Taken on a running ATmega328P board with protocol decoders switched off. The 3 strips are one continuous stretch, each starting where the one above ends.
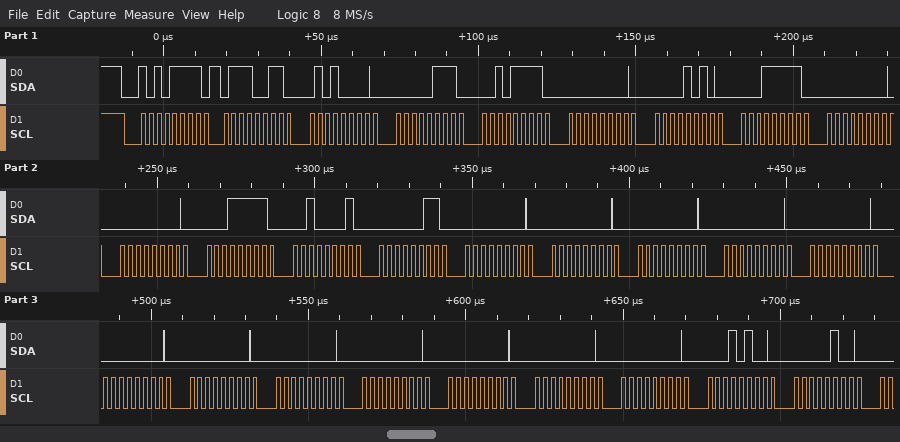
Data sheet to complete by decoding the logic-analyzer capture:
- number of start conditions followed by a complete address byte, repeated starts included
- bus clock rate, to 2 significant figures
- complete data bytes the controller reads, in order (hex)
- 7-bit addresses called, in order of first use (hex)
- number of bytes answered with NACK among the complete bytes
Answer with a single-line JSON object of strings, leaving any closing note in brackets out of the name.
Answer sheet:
{"number of start conditions followed by a complete address byte, repeated starts included": "1", "bus clock rate, to 2 significant figures": "400 kHz", "complete data bytes the controller reads, in order": "73 50 07 2F 00 0A 1F 00 00 1F 21 03 00 00 00 00 00 00 00 00 00 00 00 00 14 04", "7-bit addresses called, in order of first use": "0x57", "number of bytes answered with NACK among the complete bytes": "0"}
